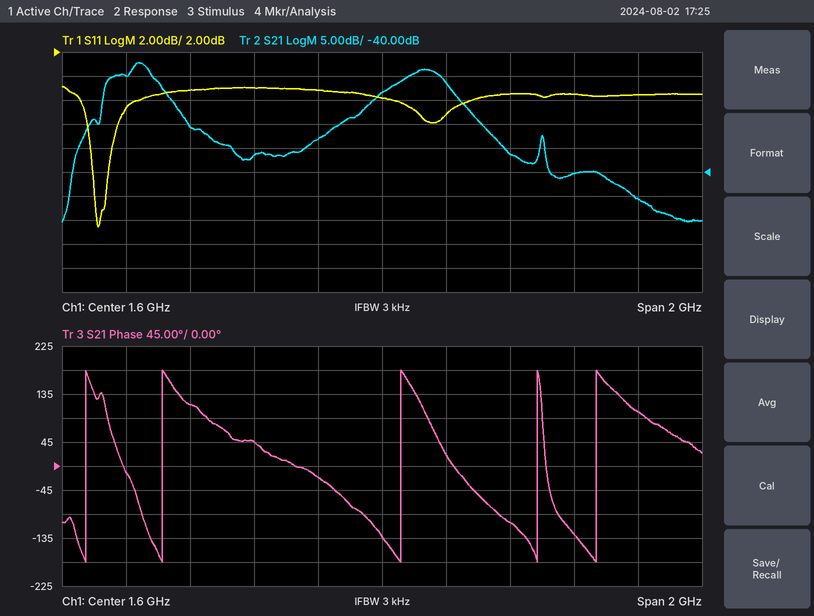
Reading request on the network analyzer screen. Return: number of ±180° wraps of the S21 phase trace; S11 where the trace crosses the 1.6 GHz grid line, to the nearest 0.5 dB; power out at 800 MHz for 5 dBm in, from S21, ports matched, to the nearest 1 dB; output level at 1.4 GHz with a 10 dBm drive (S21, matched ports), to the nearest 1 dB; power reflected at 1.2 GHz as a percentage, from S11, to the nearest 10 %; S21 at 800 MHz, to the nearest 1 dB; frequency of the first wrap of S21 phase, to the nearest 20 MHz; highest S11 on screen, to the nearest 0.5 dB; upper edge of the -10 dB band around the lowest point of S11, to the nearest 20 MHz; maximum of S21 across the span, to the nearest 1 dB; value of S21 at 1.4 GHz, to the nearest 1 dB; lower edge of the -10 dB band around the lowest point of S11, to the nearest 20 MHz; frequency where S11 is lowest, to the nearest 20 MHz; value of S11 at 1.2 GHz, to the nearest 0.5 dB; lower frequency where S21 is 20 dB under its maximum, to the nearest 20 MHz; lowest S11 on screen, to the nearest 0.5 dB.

5
-2.0 dB
-15 dBm
-23 dBm
80 %
-20 dB
680 MHz
-1.0 dB
740 MHz
-17 dB
-33 dB
700 MHz
720 MHz
-1.0 dB
640 MHz
-12.5 dB
